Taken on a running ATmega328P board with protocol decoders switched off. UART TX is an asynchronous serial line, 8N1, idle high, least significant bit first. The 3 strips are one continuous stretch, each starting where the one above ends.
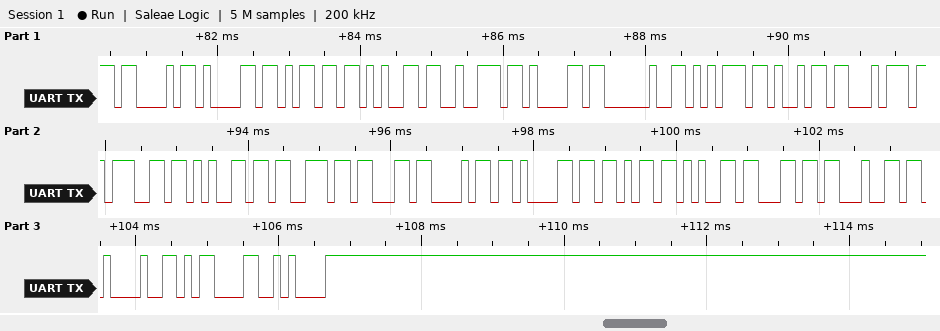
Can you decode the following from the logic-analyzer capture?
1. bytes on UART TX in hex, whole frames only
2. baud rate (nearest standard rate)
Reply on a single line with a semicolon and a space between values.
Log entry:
43 61 6D 65 72 61 20 75 69 74 67 65 73 63 68 61 6B 65 6C 64 21 0D 0A; 9600 baud
